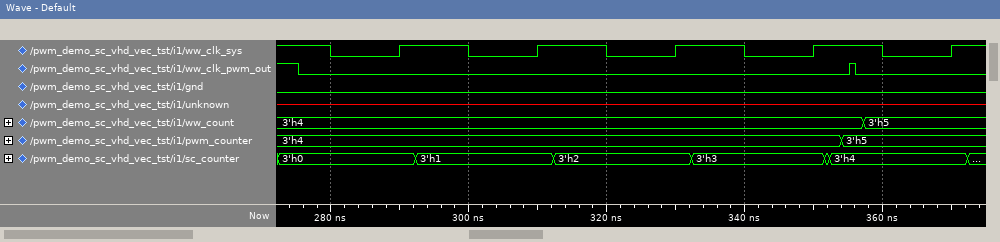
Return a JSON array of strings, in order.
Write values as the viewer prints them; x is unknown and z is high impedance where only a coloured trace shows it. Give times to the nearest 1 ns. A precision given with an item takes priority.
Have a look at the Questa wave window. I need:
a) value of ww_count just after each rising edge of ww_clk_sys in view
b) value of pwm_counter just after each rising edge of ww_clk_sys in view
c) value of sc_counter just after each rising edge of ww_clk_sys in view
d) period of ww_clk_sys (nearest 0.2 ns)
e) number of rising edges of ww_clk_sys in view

["3'h4, 3'h4, 3'h4, 3'h4, 3'h5", "3'h4, 3'h4, 3'h4, 3'h4, 3'h5", "3'h0, 3'h1, 3'h2, 3'h3, 3'h4", "20 ns", "5"]
